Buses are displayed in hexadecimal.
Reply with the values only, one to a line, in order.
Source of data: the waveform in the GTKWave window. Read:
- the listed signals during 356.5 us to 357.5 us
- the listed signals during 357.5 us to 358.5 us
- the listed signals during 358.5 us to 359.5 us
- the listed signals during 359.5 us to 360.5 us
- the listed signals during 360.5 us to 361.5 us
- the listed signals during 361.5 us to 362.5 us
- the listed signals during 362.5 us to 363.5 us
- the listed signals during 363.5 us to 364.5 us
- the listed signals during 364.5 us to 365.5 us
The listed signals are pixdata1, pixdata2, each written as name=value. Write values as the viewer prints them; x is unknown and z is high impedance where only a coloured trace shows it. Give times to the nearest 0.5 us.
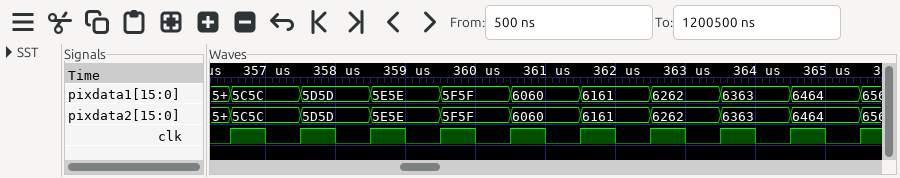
pixdata1=5C5C, pixdata2=5C5C
pixdata1=5D5D, pixdata2=5D5D
pixdata1=5E5E, pixdata2=5E5E
pixdata1=5F5F, pixdata2=5F5F
pixdata1=6060, pixdata2=6060
pixdata1=6161, pixdata2=6161
pixdata1=6262, pixdata2=6262
pixdata1=6363, pixdata2=6363
pixdata1=6464, pixdata2=6464
